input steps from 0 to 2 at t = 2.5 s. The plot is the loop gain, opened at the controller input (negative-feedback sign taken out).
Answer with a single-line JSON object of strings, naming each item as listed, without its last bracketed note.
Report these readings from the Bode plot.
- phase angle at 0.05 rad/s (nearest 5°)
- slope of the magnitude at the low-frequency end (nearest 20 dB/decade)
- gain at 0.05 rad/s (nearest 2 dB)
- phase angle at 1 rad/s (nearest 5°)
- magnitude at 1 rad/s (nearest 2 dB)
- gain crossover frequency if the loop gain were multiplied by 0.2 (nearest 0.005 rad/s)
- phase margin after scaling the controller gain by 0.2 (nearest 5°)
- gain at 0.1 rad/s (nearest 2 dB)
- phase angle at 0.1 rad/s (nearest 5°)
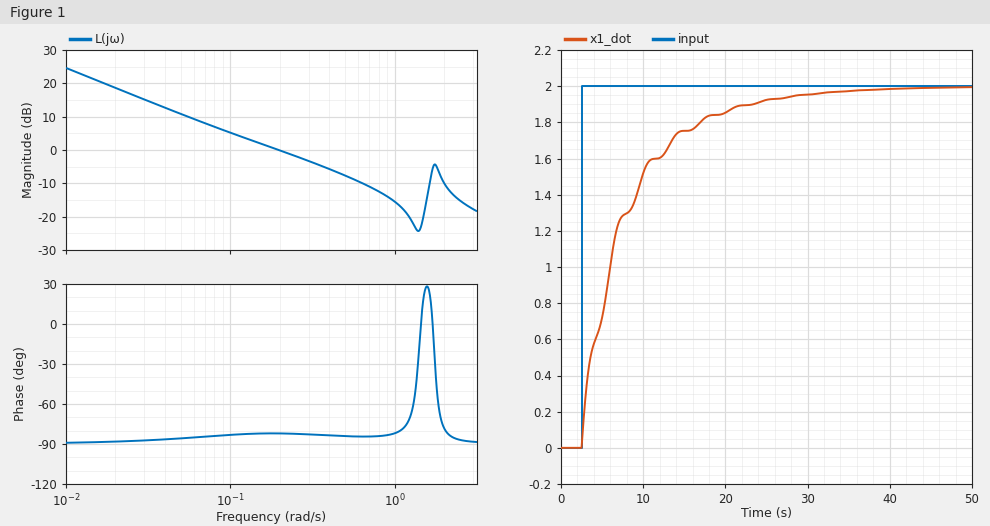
{"phase angle at 0.05 rad/s": "-85°", "slope of the magnitude at the low-frequency end": "-20 dB/decade", "gain at 0.05 rad/s": "10 dB", "phase angle at 1 rad/s": "-80°", "magnitude at 1 rad/s": "-16 dB", "gain crossover frequency if the loop gain were multiplied by 0.2": "0.035 rad/s", "phase margin after scaling the controller gain by 0.2": "95°", "gain at 0.1 rad/s": "6 dB", "phase angle at 0.1 rad/s": "-85°"}
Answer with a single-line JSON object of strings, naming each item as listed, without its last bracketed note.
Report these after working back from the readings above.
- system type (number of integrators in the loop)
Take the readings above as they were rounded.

{"system type": "1"}
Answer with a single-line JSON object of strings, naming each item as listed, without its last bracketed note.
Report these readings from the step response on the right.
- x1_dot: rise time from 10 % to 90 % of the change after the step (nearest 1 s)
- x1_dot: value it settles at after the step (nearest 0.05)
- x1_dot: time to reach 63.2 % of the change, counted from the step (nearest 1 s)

{"x1_dot: rise time from 10 % to 90 % of the change after the step": "14 s", "x1_dot: value it settles at after the step": "2.00", "x1_dot: time to reach 63.2 % of the change, counted from the step": "5 s"}
